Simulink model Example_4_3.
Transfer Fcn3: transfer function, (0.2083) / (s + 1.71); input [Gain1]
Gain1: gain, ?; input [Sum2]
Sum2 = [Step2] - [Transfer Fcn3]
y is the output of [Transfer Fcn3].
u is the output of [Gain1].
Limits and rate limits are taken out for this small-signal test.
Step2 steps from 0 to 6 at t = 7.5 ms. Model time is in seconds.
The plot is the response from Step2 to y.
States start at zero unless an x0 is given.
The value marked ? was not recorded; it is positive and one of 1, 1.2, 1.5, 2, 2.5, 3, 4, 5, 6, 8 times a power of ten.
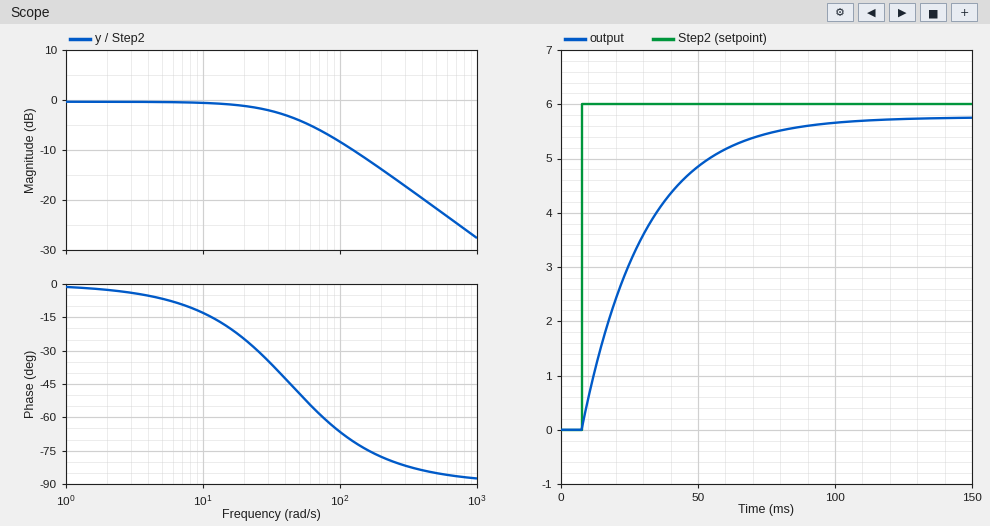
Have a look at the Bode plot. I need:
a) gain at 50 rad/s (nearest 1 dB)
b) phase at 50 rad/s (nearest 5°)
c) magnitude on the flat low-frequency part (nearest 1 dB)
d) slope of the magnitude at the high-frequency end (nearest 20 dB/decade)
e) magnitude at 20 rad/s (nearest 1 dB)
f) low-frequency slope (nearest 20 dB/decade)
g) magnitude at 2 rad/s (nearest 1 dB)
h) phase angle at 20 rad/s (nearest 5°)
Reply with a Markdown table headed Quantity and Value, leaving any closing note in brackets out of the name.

| Quantity | Value |
|---|---|
| gain at 50 rad/s | -4 dB |
| phase at 50 rad/s | -50° |
| magnitude on the flat low-frequency part | 0 dB |
| slope of the magnitude at the high-frequency end | -20 dB/decade |
| magnitude at 20 rad/s | -1 dB |
| low-frequency slope | 0 dB/decade |
| magnitude at 2 rad/s | 0 dB |
| phase angle at 20 rad/s | -25° |
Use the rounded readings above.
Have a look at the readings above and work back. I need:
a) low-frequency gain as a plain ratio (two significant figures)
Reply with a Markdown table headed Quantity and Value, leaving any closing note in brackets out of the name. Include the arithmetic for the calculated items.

| Quantity | Value |
|---|---|
| low-frequency gain as a plain ratio | 10^(0 / 20) = 1.0 |
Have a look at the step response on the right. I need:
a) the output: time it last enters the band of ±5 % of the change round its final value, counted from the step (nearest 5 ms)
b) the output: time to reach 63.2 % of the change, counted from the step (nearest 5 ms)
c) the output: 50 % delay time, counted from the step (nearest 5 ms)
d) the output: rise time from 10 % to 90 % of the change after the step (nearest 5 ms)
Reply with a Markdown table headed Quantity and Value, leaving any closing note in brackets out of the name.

| Quantity | Value |
|---|---|
| the output: time it last enters the band of ±5 % of the change round its final value, counted from the step | 70 ms |
| the output: time to reach 63.2 % of the change, counted from the step | 25 ms |
| the output: 50 % delay time, counted from the step | 15 ms |
| the output: rise time from 10 % to 90 % of the change after the step | 50 ms |
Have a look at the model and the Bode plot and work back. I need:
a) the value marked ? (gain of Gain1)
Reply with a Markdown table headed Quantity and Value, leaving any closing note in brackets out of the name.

| Quantity | Value |
|---|---|
| the value marked ? | 200 |
